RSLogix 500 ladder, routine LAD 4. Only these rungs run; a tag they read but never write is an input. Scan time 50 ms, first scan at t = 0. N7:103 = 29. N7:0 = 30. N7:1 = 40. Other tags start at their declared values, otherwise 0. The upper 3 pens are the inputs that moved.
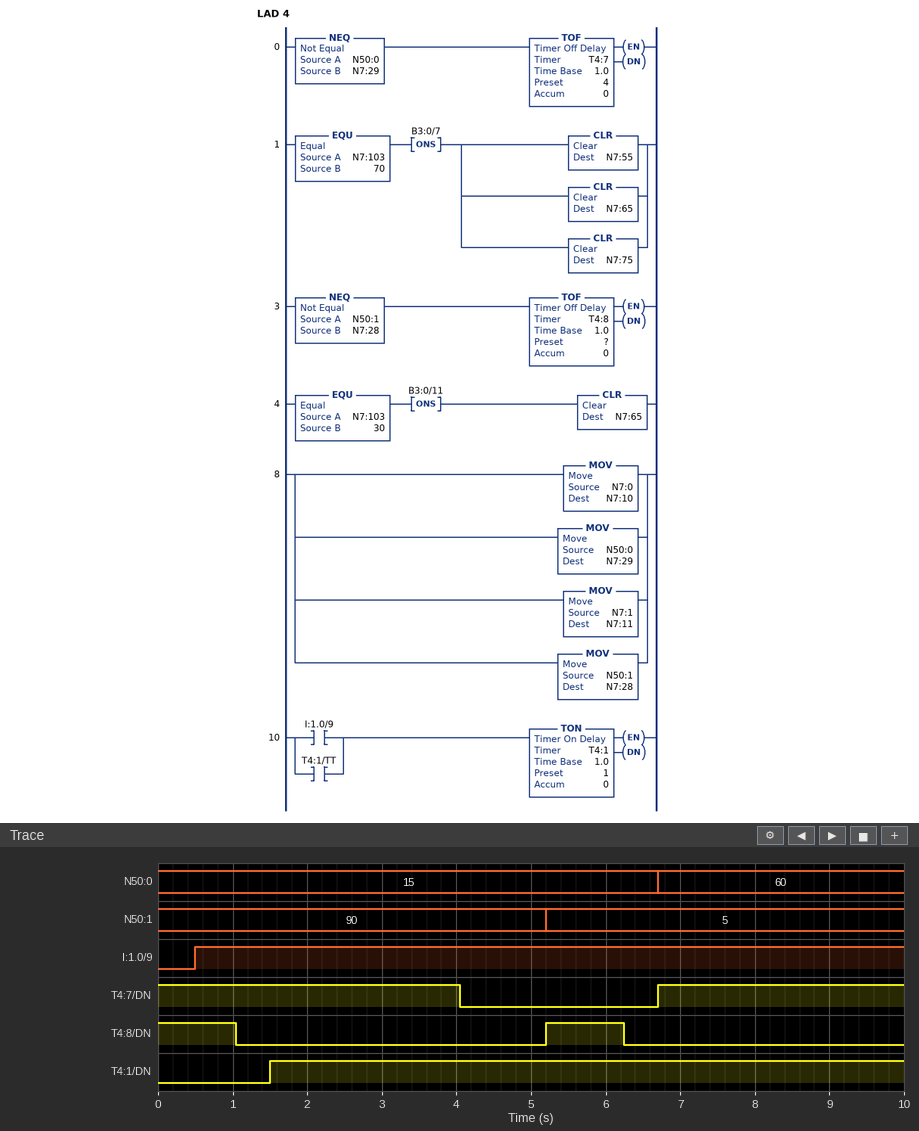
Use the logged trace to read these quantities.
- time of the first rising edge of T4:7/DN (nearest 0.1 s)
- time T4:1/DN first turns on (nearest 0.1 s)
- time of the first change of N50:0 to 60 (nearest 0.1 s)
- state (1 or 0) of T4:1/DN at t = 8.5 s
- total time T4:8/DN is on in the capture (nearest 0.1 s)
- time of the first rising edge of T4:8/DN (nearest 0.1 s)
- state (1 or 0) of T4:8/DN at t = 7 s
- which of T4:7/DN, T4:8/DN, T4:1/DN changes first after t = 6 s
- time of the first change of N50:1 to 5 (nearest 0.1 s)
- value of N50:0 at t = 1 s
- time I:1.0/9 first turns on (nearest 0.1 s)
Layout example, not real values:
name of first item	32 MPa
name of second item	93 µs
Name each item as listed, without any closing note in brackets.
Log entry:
time of the first rising edge of T4:7/DN	6.7 s
time T4:1/DN first turns on	1.5 s
time of the first change of N50:0 to 60	6.7 s
state (1 or 0) of T4:1/DN at t = 8.5 s	1
total time T4:8/DN is on in the capture	2.1 s
time of the first rising edge of T4:8/DN	5.2 s
state (1 or 0) of T4:8/DN at t = 7 s	0
which of T4:7/DN, T4:8/DN, T4:1/DN changes first after t = 6 s	T4:8/DN
time of the first change of N50:1 to 5	5.2 s
value of N50:0 at t = 1 s	15
time I:1.0/9 first turns on	0.5 s
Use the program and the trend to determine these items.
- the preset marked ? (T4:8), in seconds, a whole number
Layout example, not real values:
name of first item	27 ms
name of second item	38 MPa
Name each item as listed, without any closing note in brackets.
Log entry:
the preset marked ? (T4:8), in seconds, a whole number	1 s
